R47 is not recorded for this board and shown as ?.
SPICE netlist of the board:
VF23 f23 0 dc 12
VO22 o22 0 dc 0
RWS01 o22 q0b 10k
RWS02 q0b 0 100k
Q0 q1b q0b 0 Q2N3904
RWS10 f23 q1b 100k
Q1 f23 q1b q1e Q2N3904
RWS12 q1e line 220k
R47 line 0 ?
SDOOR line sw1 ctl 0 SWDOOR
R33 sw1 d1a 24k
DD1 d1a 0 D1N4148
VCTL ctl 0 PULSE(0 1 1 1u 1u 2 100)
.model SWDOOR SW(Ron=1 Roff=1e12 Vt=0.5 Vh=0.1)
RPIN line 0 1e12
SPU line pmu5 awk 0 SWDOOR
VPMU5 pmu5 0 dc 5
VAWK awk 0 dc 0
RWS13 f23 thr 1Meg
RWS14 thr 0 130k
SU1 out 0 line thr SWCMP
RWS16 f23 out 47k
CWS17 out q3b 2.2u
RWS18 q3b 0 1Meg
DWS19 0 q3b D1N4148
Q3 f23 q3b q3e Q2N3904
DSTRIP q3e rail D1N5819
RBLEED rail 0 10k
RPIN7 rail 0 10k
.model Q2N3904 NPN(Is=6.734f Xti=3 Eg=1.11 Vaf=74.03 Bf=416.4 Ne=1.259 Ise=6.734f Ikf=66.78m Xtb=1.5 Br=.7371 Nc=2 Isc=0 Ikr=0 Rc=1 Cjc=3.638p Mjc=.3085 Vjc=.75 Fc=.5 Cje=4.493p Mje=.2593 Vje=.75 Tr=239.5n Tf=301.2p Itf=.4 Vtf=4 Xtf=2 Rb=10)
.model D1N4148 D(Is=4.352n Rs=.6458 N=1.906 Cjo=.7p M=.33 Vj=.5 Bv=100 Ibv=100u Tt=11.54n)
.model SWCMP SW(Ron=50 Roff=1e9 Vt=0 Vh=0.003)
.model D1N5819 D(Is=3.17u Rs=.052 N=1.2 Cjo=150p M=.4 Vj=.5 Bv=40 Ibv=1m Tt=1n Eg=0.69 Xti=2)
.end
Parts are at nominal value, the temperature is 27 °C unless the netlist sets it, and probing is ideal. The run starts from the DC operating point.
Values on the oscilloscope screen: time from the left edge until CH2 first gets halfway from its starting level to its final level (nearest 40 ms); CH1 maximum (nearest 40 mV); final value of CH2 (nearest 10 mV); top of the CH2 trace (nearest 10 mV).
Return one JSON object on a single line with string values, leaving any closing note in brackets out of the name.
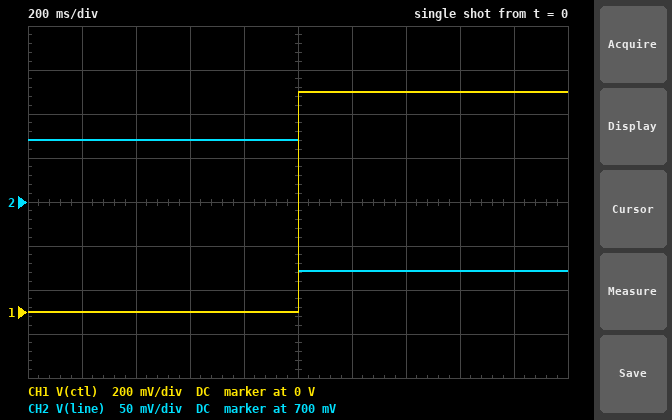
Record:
{"time from the left edge until CH2 first gets halfway from its starting level to its final level": "1.00 s", "CH1 maximum": "1.00 V", "final value of CH2": "620 mV", "top of the CH2 trace": "770 mV"}
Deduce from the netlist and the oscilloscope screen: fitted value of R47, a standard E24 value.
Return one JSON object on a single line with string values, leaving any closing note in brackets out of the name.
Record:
{"fitted value of R47, a standard E24 value": "16 kΩ"}
